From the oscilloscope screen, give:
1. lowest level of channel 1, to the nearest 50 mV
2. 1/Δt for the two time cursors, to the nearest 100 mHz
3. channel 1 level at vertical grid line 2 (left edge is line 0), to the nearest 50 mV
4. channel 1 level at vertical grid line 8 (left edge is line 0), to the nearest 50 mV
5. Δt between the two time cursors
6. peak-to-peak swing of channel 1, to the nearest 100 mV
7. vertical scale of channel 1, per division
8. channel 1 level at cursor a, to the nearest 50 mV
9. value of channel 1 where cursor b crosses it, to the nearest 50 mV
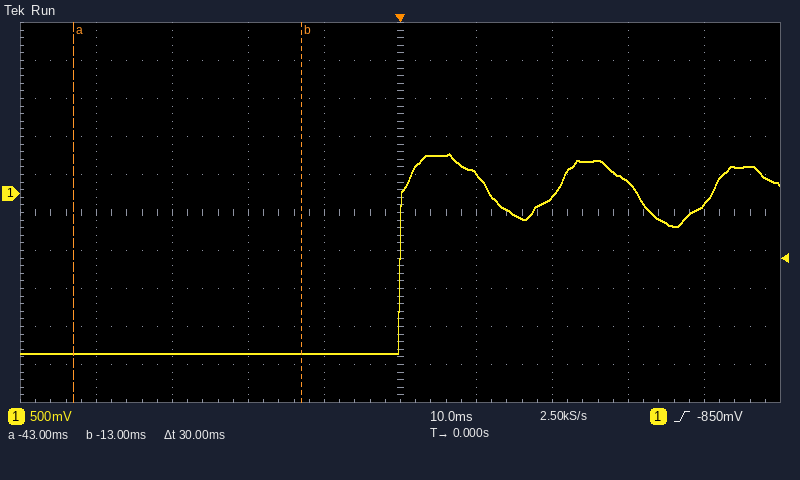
-2.10 V
33.3 Hz
-2.10 V
150 mV
30 ms
2.60 V
500 mV
-2.10 V
-2.10 V
